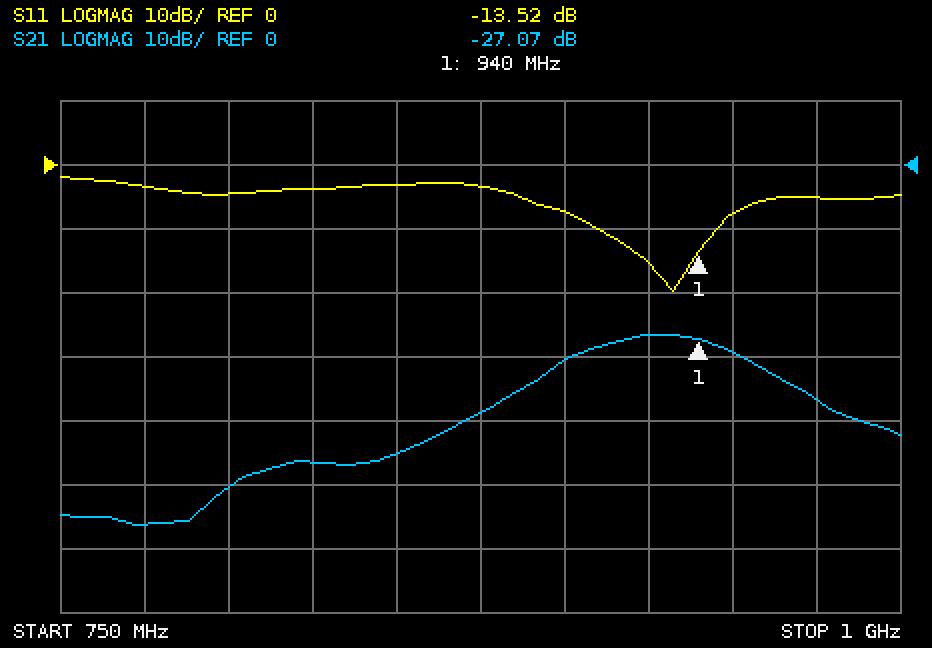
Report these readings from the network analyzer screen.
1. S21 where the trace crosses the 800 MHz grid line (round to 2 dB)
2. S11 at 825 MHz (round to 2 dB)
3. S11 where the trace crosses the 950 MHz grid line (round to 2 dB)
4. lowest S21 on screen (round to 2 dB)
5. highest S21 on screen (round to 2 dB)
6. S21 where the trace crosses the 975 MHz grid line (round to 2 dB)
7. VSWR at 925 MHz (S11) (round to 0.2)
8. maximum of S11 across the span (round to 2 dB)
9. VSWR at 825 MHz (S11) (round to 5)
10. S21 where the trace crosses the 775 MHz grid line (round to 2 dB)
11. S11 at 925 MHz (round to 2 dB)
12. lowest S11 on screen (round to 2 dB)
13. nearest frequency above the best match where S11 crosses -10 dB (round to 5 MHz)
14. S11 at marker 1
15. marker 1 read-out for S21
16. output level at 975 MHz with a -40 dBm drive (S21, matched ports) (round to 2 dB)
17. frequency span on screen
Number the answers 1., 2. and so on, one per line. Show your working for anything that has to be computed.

1. -50 dB
2. -4 dB
3. -8 dB
4. -56 dB
5. -26 dB
6. -36 dB
7. |Γ| = 10^(-16/20) = 0.1585; VSWR = (1 + 0.1585)/(1 − 0.1585) ≈ 1.4
8. -2 dB
9. |Γ| = 10^(-4/20) = 0.6310; VSWR = (1 + 0.6310)/(1 − 0.6310) ≈ 4.42, so 5 to the nearest 5
10. -56 dB
11. -16 dB
12. -20 dB
13. 945 MHz
14. -13.52 dB
15. -27.07 dB
16. -40 dBm + (-36 dB) = -76 dBm
17. 250 MHz
